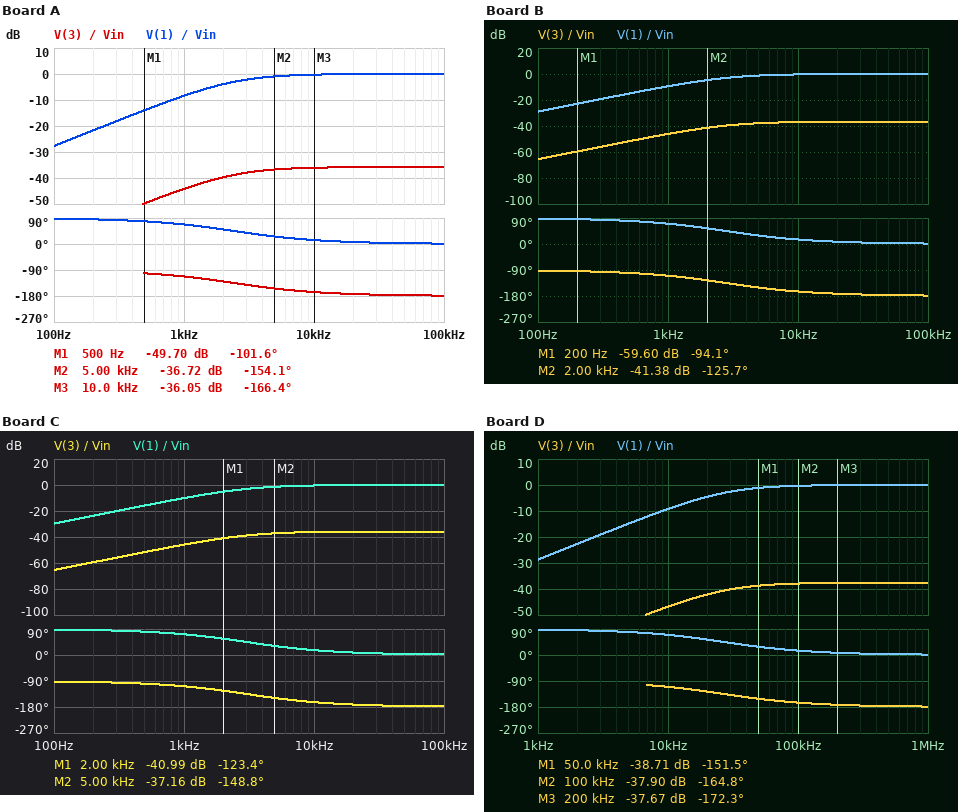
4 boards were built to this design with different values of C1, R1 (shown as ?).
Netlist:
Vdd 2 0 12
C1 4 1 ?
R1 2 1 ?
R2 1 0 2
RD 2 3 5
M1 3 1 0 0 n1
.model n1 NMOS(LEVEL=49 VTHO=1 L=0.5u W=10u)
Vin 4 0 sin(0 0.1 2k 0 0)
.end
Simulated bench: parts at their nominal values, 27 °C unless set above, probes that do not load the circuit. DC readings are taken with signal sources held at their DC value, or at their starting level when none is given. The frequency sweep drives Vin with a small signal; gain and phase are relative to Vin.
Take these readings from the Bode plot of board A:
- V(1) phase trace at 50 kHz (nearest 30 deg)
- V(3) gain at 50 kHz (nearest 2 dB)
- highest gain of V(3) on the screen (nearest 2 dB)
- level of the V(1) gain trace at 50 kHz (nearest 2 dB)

0 deg
-36 dB
-36 dB
0 dB
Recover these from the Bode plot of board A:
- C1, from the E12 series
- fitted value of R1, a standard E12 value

150 µF
0.56 Ω
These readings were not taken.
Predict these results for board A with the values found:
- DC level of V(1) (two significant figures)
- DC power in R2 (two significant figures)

9.4 V
44 W
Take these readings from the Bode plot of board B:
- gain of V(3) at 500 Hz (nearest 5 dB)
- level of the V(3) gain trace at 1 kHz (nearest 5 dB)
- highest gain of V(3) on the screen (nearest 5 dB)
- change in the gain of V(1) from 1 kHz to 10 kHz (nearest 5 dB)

-50 dB
-45 dB
-35 dB
10 dB
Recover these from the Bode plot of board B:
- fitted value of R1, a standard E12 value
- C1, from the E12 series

0.47 Ω
150 µF
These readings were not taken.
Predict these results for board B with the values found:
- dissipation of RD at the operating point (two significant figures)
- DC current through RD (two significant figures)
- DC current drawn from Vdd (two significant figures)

21 mW
65 mA
4.9 A
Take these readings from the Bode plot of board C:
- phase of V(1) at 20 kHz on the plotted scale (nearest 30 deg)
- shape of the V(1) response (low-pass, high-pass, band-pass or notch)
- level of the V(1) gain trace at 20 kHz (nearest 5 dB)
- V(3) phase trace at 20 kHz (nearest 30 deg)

0 deg
high-pass
0 dB
-180 deg
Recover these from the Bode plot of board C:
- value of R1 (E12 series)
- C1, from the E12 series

0.56 Ω
120 µF
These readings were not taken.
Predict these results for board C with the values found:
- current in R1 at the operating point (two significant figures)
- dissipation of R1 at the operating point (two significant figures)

4.7 A
12 W
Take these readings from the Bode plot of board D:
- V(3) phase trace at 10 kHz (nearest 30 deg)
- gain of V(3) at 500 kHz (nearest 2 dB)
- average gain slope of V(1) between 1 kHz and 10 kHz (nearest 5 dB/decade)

-120 deg
-38 dB
20 dB/decade
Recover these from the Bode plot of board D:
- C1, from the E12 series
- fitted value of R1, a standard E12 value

18 µF
0.39 Ω
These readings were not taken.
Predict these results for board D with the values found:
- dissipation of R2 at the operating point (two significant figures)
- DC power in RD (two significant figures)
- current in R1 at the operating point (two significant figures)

50 W
22 mW
5.0 A
